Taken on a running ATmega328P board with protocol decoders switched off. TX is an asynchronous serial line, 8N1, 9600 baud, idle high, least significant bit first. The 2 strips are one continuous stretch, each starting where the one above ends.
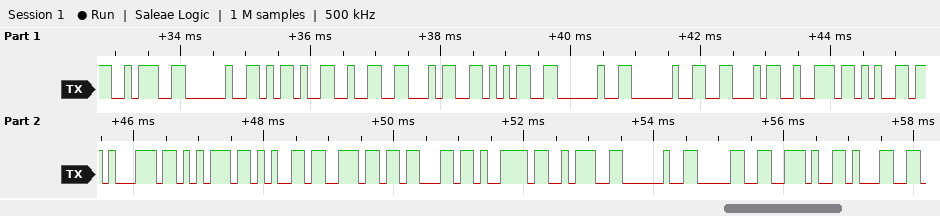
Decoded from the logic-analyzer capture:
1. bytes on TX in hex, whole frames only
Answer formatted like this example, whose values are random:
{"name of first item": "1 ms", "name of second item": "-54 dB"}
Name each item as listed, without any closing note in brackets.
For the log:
{"bytes on TX in hex, whole frames only": "3A 20 2D 32 34 35 20 20 46 72 65 71 75 65 6E 63 79 3A 20 30 2E 31"}
